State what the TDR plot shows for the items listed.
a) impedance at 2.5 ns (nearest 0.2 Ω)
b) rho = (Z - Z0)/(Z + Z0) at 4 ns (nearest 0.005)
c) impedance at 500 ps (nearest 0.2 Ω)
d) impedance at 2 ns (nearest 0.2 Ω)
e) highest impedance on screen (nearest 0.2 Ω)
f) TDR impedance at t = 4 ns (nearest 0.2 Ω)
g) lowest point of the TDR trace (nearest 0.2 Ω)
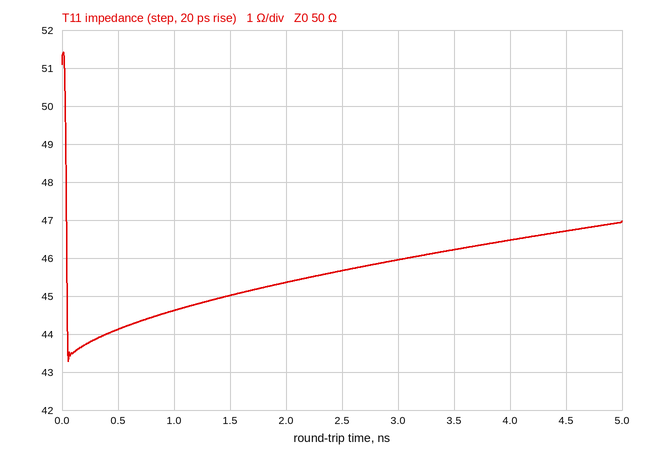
45.6 Ω
-0.035
44.2 Ω
45.4 Ω
51.4 Ω
46.4 Ω
43.2 Ω
